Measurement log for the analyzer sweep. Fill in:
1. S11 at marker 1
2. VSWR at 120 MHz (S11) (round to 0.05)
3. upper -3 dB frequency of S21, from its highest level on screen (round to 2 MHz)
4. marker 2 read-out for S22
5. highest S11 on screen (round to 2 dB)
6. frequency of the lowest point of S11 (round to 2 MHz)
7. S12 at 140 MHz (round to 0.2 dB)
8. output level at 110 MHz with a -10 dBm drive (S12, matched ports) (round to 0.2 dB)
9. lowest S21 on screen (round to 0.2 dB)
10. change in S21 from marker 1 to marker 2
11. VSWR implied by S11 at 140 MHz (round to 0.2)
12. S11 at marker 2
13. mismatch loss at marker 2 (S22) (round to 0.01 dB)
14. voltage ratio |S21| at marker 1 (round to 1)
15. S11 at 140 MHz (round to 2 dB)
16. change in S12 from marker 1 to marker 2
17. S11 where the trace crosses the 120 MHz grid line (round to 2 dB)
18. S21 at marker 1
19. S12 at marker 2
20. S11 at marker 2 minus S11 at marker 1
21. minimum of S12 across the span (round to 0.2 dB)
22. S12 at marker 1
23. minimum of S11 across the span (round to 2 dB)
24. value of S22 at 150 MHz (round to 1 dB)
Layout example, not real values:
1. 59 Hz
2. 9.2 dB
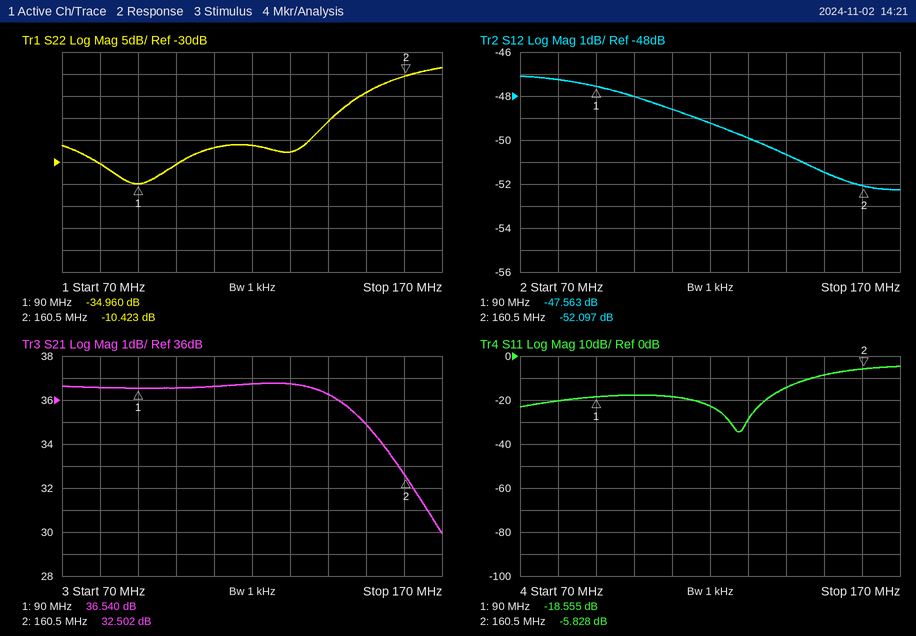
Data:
1. -18.555 dB
2. 1.15
3. 156 MHz
4. -10.423 dB
5. -4 dB
6. 128 MHz
7. -50.6 dB
8. -58.6 dBm
9. 30.0 dB
10. -4.038 dB
11. 1.4
12. -5.828 dB
13. 0.41 dB
14. 67
15. -14 dB
16. -4.534 dB
17. -22 dB
18. 36.540 dB
19. -52.097 dB
20. 12.727 dB
21. -52.2 dB
22. -47.563 dB
23. -34 dB
24. -14 dB
